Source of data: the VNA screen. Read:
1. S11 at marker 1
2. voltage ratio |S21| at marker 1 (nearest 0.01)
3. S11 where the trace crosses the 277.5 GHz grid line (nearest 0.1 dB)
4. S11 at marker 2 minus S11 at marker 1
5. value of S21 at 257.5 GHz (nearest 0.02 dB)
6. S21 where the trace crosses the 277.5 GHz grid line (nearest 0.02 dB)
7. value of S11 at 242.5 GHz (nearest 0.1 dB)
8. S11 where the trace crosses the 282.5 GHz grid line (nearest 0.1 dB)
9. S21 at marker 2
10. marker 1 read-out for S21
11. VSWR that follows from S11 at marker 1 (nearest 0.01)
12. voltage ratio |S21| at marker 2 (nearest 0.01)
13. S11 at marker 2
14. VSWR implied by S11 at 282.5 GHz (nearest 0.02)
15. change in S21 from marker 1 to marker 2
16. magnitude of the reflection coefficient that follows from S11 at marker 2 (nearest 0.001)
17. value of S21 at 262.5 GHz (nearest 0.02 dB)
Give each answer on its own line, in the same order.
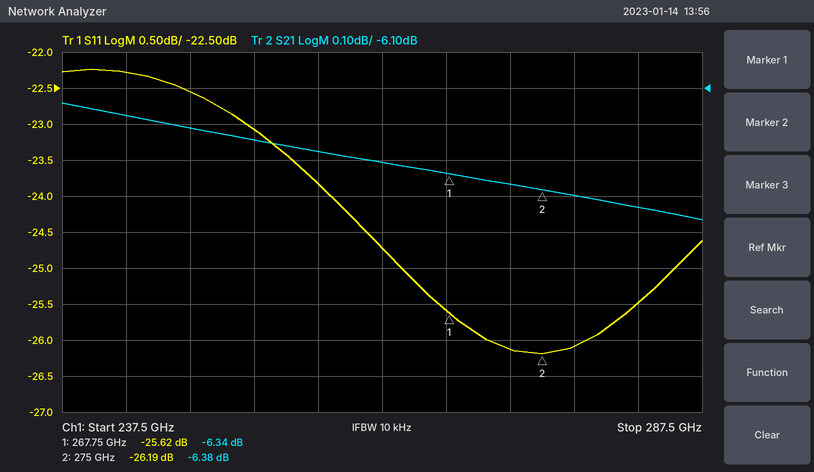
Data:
-25.62 dB
0.48
-26.1 dB
-0.57 dB
-6.28 dB
-6.40 dB
-22.3 dB
-25.5 dB
-6.38 dB
-6.34 dB
1.11
0.48
-26.19 dB
1.12
-0.04 dB
0.049
-6.30 dB
